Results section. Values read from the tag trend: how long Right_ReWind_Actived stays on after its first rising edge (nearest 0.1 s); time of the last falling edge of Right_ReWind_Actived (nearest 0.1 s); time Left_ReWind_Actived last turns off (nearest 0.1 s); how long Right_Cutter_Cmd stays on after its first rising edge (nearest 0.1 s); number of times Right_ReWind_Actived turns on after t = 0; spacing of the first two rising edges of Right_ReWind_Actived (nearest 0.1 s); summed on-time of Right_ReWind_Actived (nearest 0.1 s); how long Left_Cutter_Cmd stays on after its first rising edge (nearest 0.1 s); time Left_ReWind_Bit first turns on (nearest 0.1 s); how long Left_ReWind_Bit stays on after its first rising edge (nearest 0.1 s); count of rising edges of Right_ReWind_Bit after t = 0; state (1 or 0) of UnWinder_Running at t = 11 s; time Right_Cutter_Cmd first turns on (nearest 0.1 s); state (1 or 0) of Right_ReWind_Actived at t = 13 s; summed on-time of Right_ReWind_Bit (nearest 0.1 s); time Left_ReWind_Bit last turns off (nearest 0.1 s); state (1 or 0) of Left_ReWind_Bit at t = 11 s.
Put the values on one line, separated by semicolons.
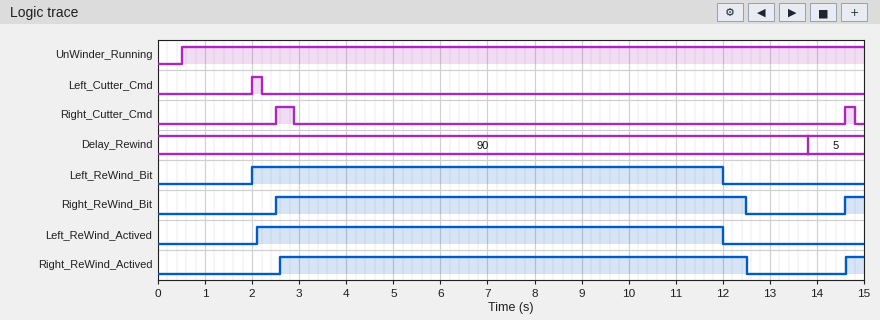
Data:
9.9 s; 12.5 s; 12.0 s; 0.4 s; 2; 12.0 s; 10.3 s; 0.2 s; 2.0 s; 10.0 s; 2; 1; 2.5 s; 0; 10.4 s; 12.0 s; 1
